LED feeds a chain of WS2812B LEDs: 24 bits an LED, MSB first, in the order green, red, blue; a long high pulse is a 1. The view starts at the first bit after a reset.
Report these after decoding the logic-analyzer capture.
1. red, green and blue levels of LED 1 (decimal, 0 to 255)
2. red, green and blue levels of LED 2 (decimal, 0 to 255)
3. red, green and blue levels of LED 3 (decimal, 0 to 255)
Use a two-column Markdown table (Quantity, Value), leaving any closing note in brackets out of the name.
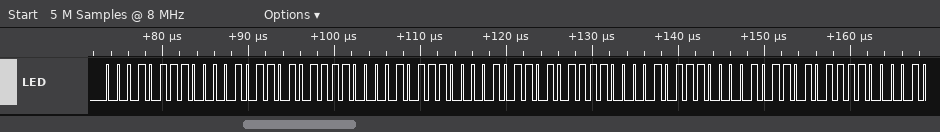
| Quantity | Value |
|---|---|
| red, green and blue levels of LED 1 | 11, 23, 94 |
| red, green and blue levels of LED 2 | 11, 23, 94 |
| red, green and blue levels of LED 3 | 11, 23, 94 |
